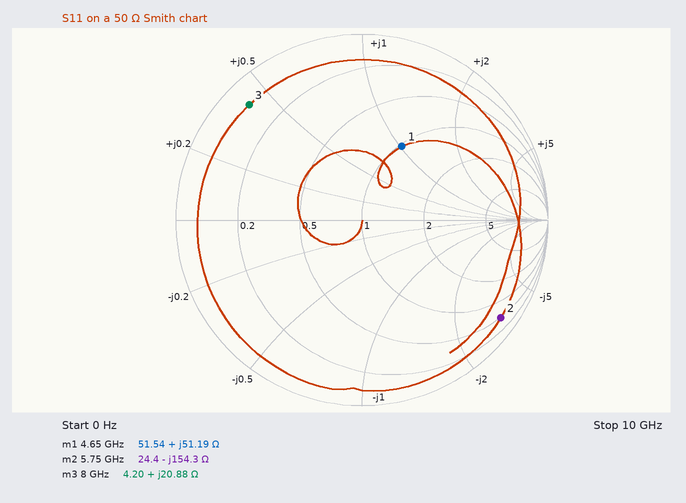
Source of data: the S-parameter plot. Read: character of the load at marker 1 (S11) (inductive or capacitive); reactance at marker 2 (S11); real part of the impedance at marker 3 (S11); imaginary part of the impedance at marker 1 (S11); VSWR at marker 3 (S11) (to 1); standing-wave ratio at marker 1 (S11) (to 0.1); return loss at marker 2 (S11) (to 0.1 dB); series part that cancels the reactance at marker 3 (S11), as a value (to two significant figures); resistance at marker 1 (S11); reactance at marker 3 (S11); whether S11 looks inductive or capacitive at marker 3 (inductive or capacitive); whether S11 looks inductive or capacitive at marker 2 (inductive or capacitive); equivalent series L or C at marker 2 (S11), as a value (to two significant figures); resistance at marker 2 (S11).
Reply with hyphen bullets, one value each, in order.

- inductive
- -154.3 Ω
- 4.20 Ω
- +51.19 Ω
- 14
- 2.6
- 0.8 dB
- 950 fF
- 51.54 Ω
- +20.88 Ω
- inductive
- capacitive
- 180 fF
- 24.4 Ω
